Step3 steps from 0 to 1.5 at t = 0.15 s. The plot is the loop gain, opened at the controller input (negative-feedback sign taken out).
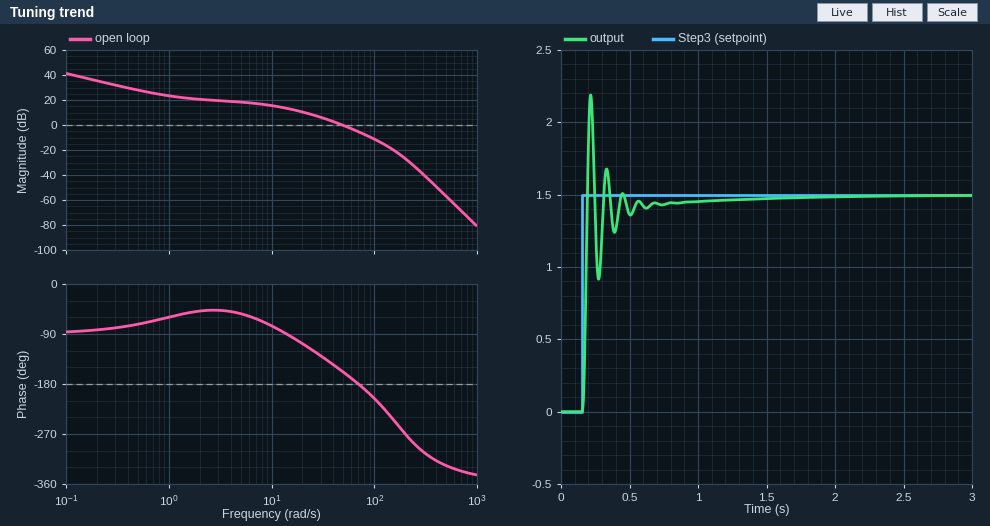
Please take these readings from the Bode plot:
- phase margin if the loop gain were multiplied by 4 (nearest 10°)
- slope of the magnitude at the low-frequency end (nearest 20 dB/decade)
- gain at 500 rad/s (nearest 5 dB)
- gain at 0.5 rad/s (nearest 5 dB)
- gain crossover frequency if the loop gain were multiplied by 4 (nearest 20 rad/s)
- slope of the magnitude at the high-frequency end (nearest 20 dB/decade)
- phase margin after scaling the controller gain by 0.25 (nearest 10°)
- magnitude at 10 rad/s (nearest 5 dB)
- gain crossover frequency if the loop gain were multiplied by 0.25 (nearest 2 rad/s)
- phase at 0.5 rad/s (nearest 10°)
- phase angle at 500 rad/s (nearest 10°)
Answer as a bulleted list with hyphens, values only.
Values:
- -30°
- -20 dB/decade
- -55 dB
- 30 dB
- 100 rad/s
- -80 dB/decade
- 80°
- 15 dB
- 16 rad/s
- -70°
- -330°
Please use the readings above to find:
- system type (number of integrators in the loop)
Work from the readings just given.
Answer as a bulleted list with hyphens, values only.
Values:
- 1
